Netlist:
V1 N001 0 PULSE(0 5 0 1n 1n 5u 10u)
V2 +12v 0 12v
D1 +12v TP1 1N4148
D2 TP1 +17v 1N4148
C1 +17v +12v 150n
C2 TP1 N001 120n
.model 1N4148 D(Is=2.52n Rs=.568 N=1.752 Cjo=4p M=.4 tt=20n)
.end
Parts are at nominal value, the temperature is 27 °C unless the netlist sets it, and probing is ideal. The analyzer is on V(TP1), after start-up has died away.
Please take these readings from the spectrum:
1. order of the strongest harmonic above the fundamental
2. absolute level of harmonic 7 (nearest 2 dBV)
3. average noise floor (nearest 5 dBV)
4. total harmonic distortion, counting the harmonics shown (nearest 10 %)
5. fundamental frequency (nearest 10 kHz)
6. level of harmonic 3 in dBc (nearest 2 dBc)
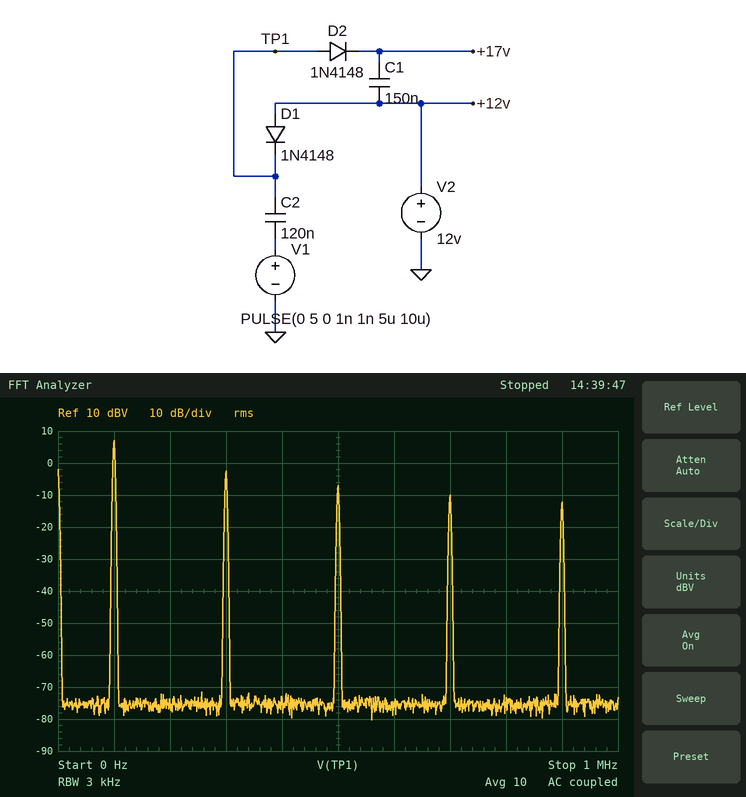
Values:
3
-10 dBV
-75 dBV
40 %
100 kHz
-10 dBc
